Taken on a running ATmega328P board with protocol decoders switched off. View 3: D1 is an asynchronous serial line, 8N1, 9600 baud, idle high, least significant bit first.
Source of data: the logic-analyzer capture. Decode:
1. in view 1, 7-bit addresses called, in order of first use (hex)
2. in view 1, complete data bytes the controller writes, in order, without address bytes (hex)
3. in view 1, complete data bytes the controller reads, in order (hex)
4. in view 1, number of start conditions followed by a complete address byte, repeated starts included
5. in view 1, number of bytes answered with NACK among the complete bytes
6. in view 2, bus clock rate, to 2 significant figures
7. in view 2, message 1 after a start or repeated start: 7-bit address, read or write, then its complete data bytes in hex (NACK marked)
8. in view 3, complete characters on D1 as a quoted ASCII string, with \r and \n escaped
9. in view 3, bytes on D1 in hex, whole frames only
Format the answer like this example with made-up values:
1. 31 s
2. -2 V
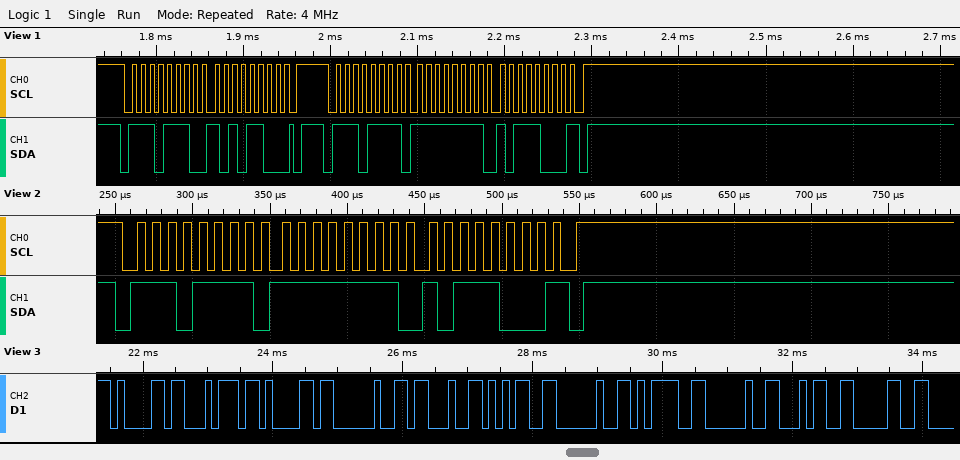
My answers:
1. 0x77
2. AC
3. FF B8
4. 2
5. 1
6. 100 kHz
7. 0x77 read: FF B8 NACK
8. "ata #5 = 40"
9. 61 74 61 20 23 35 20 3D 20 34 30
